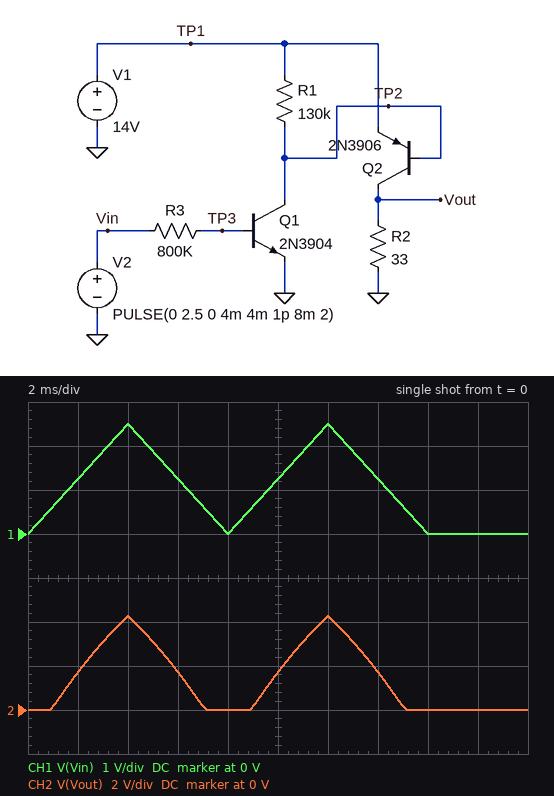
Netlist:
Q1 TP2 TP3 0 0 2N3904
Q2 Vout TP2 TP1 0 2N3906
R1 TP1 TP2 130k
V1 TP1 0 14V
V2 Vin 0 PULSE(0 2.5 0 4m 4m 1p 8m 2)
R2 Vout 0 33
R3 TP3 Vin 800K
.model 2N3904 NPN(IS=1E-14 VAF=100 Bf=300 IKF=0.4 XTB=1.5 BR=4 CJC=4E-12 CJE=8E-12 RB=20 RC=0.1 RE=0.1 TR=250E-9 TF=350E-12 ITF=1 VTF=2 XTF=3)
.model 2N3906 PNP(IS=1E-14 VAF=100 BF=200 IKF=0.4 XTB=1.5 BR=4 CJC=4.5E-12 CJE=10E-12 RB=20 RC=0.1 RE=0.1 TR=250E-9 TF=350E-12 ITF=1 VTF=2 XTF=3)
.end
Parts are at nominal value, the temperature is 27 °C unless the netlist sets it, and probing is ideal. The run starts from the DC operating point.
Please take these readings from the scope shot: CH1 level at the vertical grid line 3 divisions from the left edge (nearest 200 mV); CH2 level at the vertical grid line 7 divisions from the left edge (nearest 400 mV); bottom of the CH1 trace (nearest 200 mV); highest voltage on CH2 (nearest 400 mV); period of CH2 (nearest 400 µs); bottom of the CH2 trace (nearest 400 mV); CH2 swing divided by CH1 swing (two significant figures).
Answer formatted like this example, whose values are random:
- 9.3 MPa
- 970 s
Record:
- 1.2 V
- 1.6 V
- 0 V
- 4.4 V
- 8.0 ms
- 0 V
- 1.7
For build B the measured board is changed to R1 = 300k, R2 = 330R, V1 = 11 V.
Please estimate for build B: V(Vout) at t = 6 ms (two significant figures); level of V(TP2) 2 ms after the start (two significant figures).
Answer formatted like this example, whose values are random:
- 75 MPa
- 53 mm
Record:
- 11 V
- 10 V
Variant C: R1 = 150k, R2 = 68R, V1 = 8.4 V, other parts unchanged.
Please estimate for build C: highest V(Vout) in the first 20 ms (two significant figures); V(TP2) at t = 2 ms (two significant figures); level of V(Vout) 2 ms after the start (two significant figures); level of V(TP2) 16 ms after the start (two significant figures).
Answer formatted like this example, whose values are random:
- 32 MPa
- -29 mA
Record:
- 7.8 V
- 7.6 V
- 3.2 V
- 8.4 V
